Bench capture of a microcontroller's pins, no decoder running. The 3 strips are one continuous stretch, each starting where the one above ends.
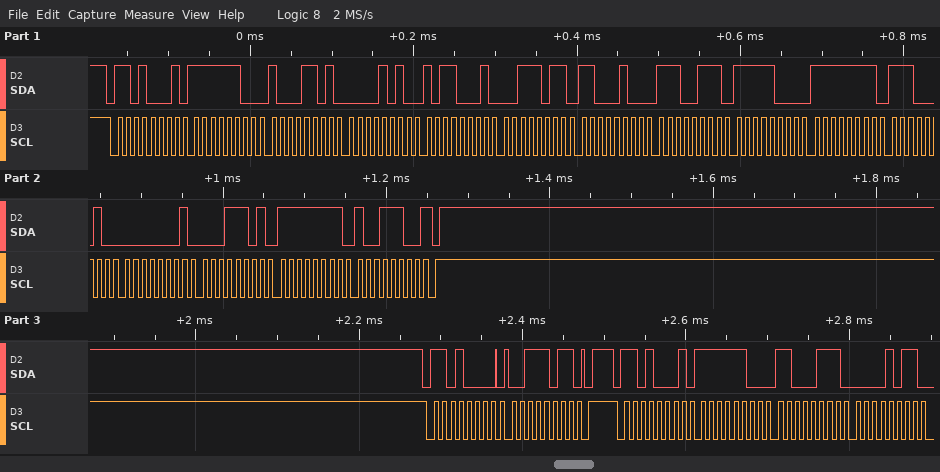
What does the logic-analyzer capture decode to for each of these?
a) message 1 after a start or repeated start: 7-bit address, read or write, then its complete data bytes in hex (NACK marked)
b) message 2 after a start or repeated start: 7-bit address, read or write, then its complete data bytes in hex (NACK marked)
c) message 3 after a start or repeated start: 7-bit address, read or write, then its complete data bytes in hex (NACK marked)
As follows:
0x68 read: FC 8D 0A B1 3B C4 E7 F8 FF E2 01 1D FF 9C NACK
0x68 write: 3B
0x68 read: FC C7 0B
